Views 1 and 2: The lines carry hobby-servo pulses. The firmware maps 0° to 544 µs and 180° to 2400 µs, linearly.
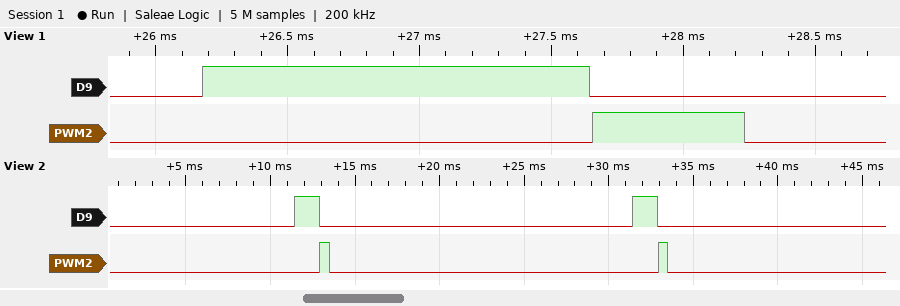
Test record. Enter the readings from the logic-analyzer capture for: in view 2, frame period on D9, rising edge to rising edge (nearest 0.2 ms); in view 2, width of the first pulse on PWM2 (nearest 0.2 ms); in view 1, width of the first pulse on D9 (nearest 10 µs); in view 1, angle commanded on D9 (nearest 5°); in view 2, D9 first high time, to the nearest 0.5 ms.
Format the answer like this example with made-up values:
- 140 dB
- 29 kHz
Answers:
- 20.0 ms
- 0.6 ms
- 1470 µs
- 90°
- 1.5 ms
